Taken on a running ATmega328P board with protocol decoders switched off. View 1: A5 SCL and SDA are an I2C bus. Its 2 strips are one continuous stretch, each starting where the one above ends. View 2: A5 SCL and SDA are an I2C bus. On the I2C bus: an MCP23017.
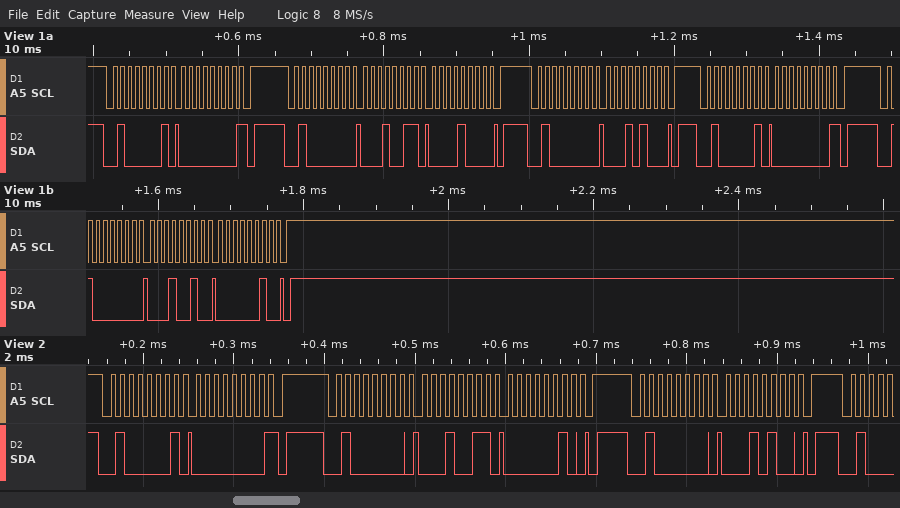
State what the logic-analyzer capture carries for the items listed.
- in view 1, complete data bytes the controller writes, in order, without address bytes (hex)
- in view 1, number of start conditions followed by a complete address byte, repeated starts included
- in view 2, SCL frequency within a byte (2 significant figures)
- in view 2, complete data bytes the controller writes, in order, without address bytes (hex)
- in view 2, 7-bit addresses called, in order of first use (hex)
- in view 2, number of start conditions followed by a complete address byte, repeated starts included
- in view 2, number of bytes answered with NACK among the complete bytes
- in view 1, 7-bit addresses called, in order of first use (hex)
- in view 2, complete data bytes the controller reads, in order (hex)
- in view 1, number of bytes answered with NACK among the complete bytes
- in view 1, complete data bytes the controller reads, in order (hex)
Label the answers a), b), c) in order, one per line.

a) 13 08 14 12 02
b) 5
c) 100 kHz
d) 13 02 14
e) 0x20
f) 3
g) 1
h) 0x20
i) 00
j) 2
k) 00 00
